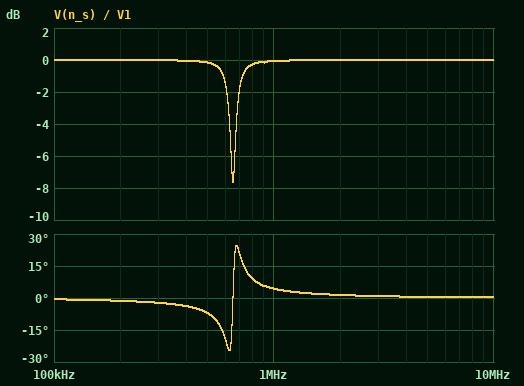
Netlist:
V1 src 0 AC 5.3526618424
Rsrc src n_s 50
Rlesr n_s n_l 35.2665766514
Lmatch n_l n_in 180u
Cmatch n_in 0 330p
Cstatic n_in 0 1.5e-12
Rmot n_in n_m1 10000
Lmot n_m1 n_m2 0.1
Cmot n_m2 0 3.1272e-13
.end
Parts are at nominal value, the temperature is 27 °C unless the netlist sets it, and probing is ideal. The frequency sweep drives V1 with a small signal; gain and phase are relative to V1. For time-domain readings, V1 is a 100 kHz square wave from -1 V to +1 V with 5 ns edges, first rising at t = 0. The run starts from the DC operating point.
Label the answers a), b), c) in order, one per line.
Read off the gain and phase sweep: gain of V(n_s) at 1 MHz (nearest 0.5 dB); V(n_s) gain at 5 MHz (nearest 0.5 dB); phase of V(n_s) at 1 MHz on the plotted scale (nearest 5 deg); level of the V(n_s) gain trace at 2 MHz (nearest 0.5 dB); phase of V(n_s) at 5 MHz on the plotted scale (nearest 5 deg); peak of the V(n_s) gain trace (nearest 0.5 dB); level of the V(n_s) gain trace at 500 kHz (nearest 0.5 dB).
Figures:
a) 0 dB
b) 0 dB
c) 5 deg
d) 0 dB
e) 0 deg
f) 0 dB
g) 0 dB
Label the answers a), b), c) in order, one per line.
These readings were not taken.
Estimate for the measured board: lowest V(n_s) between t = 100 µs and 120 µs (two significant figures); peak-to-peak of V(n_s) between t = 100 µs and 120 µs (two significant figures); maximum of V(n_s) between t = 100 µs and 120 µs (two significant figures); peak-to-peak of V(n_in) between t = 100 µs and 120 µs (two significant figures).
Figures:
a) -1.1 V
b) 2.2 V
c) 1.1 V
d) 5.1 V
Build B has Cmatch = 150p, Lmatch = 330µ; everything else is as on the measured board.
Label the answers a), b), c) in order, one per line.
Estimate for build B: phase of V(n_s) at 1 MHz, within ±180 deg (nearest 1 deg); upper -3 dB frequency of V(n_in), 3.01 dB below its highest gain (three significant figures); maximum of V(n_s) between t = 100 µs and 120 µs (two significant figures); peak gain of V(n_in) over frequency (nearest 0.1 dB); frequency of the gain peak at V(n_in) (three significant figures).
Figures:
a) 3 deg
b) 729 kHz
c) 1.1 V
d) 24.7 dB
e) 709 kHz
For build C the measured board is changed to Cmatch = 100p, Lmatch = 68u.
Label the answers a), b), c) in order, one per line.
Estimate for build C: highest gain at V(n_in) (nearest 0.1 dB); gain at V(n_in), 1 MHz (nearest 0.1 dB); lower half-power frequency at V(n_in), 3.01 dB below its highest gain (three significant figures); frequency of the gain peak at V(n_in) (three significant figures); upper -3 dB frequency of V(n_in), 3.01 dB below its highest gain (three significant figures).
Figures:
a) 19.7 dB
b) 2.7 dB
c) 1.81 MHz
d) 1.91 MHz
e) 2.01 MHz
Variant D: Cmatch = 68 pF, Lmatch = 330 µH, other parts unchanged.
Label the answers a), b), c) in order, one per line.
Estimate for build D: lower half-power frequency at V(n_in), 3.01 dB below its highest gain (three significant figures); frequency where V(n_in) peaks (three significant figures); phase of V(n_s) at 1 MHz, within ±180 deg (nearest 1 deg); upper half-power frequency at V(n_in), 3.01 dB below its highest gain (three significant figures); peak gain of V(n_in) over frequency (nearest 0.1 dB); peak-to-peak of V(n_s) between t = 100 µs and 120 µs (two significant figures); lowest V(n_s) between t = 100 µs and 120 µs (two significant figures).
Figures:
a) 1.04 MHz
b) 1.06 MHz
c) -10 deg
d) 1.08 MHz
e) 28.1 dB
f) 2.1 V
g) -1.0 V
